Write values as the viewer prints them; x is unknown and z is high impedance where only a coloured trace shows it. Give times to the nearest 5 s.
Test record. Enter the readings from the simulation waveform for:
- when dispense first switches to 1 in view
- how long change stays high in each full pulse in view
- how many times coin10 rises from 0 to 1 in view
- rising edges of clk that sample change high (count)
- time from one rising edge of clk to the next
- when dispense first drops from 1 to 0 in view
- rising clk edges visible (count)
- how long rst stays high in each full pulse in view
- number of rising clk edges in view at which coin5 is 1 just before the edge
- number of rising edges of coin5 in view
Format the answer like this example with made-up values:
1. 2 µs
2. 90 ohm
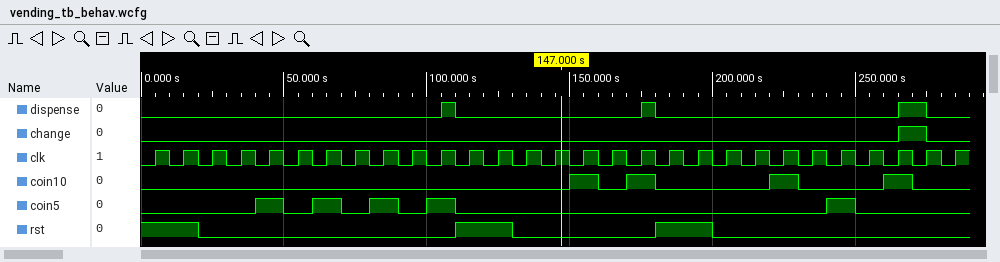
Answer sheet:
1. 105 s
2. 10 s
3. 4
4. 1
5. 10 s
6. 110 s
7. 29
8. 20 s, 20 s
9. 5
10. 5
